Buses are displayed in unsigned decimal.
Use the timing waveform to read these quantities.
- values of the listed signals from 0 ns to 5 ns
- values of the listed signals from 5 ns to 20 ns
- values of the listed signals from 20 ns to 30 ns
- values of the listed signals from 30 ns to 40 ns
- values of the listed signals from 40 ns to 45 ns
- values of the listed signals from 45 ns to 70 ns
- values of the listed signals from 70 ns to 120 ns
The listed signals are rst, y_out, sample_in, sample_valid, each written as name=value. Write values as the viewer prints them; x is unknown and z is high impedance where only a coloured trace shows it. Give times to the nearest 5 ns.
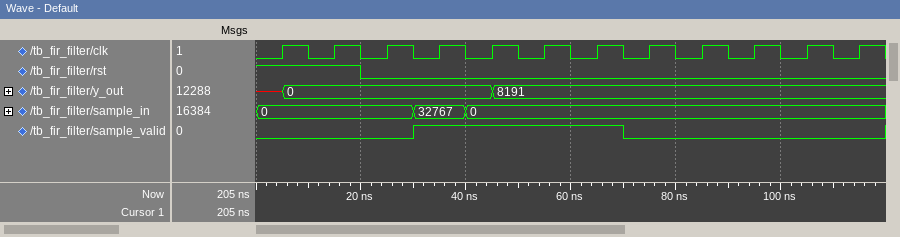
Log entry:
rst=1, y_out=x, sample_in=0, sample_valid=0
rst=1, y_out=0, sample_in=0, sample_valid=0
rst=0, y_out=0, sample_in=0, sample_valid=0
rst=0, y_out=0, sample_in=32767, sample_valid=1
rst=0, y_out=0, sample_in=0, sample_valid=1
rst=0, y_out=8191, sample_in=0, sample_valid=1
rst=0, y_out=8191, sample_in=0, sample_valid=0
